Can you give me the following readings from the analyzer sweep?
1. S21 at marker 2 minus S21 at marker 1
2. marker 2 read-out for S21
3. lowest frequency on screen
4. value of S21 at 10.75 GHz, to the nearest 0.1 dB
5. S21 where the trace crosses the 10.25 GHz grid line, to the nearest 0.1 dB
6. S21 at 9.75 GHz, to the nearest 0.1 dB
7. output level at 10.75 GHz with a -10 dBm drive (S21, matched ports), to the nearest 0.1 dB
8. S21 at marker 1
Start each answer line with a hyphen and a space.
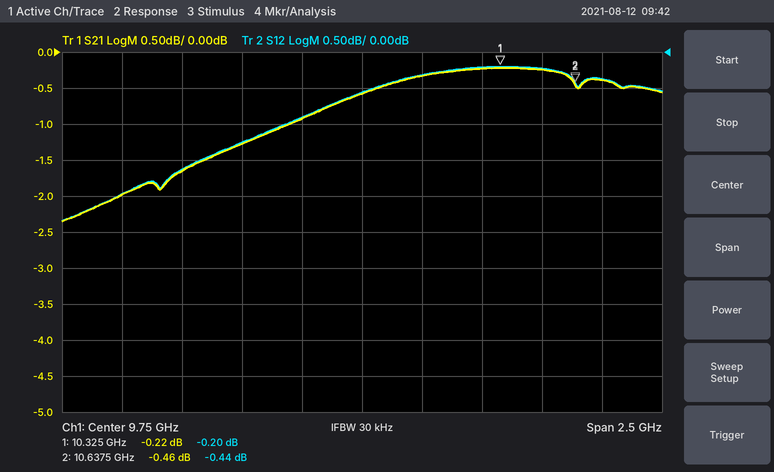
- -0.24 dB
- -0.46 dB
- 8.5 GHz
- -0.4 dB
- -0.2 dB
- -0.6 dB
- -10.4 dBm
- -0.22 dB
